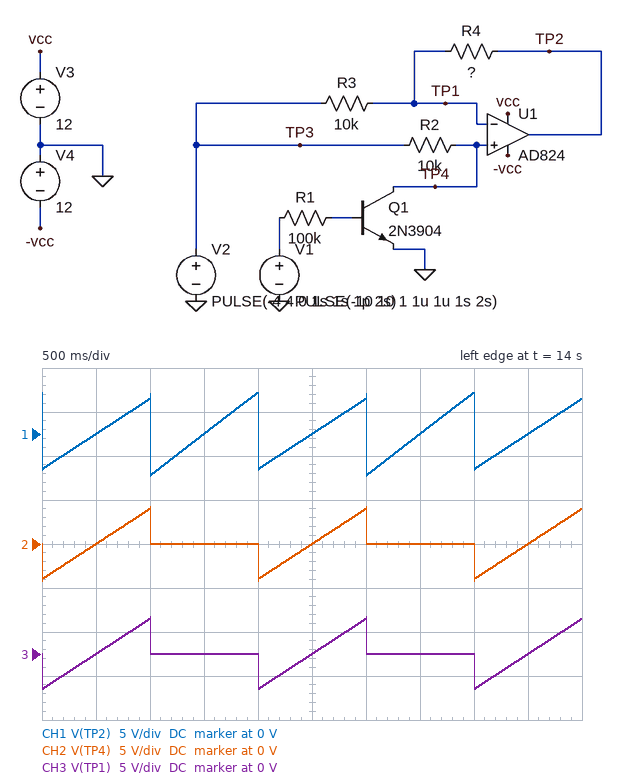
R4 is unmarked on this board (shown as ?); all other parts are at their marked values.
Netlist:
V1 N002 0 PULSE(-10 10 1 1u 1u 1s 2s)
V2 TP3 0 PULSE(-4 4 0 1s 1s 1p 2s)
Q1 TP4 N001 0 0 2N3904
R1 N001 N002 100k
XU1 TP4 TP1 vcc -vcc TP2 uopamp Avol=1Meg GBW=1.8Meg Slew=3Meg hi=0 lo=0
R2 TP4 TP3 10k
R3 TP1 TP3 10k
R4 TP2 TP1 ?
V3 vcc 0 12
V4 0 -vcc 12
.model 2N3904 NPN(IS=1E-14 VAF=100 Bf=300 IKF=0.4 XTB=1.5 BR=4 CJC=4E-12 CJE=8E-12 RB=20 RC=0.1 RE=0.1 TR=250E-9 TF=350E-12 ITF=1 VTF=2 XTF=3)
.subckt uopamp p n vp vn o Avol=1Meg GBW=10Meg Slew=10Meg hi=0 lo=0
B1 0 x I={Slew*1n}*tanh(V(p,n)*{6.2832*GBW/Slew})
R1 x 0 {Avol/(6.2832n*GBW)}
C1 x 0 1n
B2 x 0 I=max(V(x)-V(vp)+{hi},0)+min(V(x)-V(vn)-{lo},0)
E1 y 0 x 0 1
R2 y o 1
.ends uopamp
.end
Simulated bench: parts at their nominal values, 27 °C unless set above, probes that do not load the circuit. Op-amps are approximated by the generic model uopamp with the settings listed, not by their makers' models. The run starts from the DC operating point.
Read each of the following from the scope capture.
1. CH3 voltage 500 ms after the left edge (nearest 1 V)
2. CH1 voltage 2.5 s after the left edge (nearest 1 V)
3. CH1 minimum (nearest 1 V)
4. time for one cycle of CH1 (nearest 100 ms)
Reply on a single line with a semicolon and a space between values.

0 V; 0 V; -5 V; 1.0 s
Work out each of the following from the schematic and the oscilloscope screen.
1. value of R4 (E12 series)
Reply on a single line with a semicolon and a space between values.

12 kΩ
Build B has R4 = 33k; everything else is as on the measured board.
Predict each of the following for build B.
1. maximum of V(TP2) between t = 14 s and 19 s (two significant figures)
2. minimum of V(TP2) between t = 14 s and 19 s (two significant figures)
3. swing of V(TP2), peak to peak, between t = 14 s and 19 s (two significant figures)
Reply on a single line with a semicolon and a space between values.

12 V; -12 V; 24 V
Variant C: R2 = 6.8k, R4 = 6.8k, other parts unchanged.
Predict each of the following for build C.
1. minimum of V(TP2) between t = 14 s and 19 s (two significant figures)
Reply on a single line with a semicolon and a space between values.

-4.1 V
